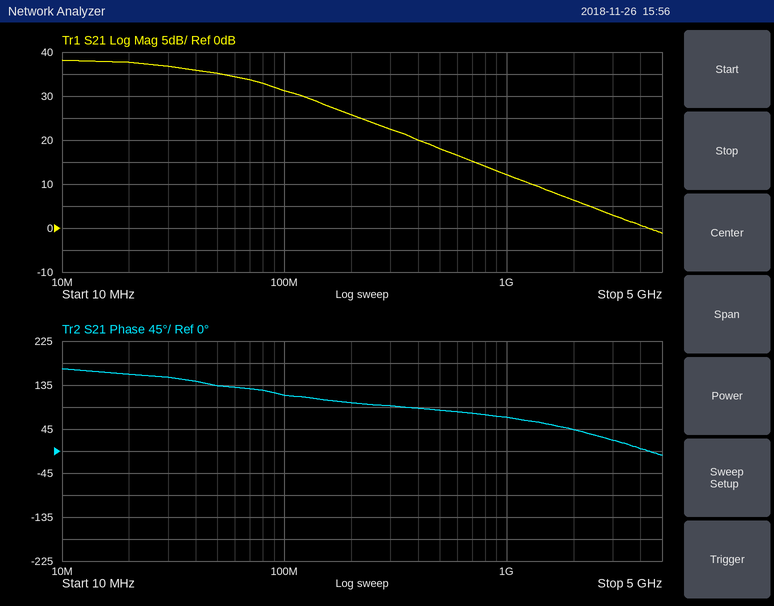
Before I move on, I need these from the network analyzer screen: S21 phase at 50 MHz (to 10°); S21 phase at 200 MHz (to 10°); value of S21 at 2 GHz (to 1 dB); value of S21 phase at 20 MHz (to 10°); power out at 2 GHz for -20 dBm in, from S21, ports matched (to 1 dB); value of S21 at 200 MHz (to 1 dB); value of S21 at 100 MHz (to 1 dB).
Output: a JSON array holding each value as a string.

["130°", "100°", "6 dB", "160°", "-14 dBm", "26 dB", "31 dB"]
